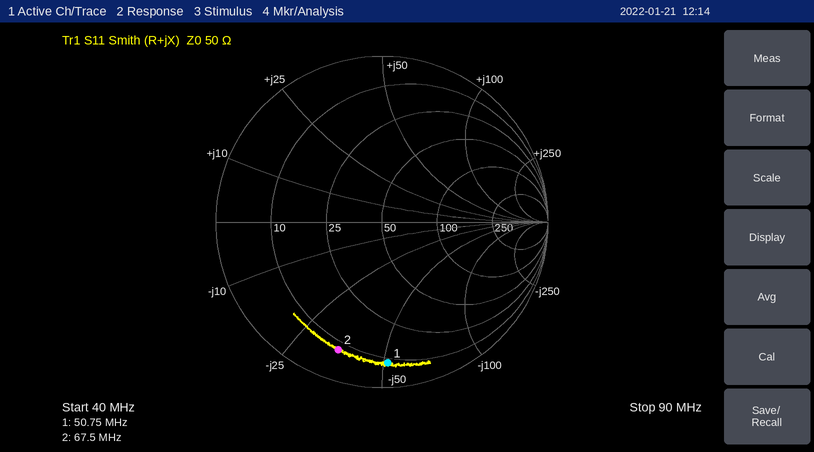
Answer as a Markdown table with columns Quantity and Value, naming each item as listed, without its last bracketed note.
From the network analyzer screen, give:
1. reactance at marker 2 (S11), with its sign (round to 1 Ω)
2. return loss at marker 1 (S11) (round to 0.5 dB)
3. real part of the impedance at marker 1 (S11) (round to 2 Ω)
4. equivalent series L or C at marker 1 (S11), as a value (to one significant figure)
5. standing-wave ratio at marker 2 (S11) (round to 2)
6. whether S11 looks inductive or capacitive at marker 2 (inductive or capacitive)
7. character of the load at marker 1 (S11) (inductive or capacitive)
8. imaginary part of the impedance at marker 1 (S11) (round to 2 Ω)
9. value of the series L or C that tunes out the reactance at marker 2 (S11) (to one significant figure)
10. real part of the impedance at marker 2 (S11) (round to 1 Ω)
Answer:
| Quantity | Value |
|---|---|
| reactance at marker 2 (S11), with its sign | -35 Ω |
| return loss at marker 1 (S11) | 1.5 dB |
| real part of the impedance at marker 1 (S11) | 8 Ω |
| equivalent series L or C at marker 1 (S11), as a value | 60 pF |
| standing-wave ratio at marker 2 (S11) | 10 |
| whether S11 looks inductive or capacitive at marker 2 | capacitive |
| character of the load at marker 1 (S11) | capacitive |
| imaginary part of the impedance at marker 1 (S11) | -52 Ω |
| value of the series L or C that tunes out the reactance at marker 2 (S11) | 80 nH |
| real part of the impedance at marker 2 (S11) | 8 Ω |
